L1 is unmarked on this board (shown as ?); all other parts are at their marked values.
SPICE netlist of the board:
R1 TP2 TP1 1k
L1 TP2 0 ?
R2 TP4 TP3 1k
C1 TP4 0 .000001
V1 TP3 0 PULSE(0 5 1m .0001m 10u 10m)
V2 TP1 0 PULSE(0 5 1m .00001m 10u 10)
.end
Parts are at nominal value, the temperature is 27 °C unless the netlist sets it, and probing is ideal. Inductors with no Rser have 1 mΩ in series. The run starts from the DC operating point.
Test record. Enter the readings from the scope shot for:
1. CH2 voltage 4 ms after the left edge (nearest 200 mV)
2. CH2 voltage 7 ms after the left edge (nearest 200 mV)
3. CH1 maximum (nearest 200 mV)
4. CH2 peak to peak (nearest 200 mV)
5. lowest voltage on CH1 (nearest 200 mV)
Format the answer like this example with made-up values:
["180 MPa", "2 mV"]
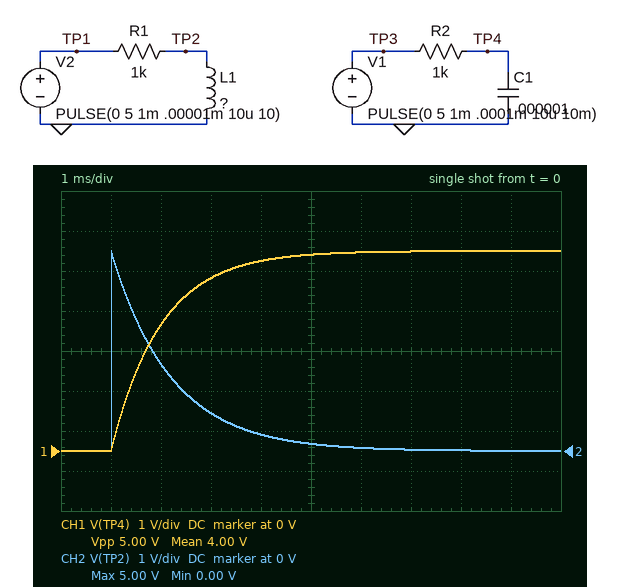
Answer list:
["400 mV", "0 V", "5.0 V", "5.0 V", "0 V"]
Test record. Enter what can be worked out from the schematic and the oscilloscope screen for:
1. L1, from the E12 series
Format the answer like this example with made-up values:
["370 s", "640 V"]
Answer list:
["1.2 H"]
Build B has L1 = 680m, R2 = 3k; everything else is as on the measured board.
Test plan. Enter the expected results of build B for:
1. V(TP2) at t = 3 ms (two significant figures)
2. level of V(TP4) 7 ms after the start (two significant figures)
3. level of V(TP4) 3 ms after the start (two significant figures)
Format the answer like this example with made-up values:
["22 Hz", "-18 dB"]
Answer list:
["260 mV", "4.3 V", "2.4 V"]
